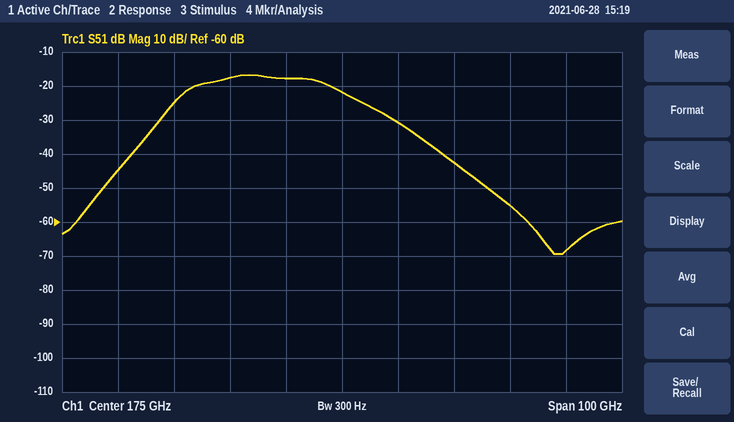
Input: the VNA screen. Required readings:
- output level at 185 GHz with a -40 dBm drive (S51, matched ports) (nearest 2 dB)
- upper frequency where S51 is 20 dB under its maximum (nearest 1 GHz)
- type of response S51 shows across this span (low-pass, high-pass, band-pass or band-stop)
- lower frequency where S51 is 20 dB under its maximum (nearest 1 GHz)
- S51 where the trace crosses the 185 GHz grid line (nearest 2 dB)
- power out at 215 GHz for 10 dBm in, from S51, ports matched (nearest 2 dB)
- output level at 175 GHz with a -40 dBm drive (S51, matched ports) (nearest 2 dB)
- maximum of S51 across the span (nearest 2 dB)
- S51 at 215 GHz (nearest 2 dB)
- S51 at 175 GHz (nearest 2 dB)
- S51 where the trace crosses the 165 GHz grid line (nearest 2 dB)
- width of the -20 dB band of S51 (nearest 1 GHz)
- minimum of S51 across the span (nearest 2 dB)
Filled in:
-70 dBm
190 GHz
band-pass
139 GHz
-30 dB
-58 dBm
-62 dBm
-16 dB
-68 dB
-22 dB
-18 dB
51 GHz
-70 dB
